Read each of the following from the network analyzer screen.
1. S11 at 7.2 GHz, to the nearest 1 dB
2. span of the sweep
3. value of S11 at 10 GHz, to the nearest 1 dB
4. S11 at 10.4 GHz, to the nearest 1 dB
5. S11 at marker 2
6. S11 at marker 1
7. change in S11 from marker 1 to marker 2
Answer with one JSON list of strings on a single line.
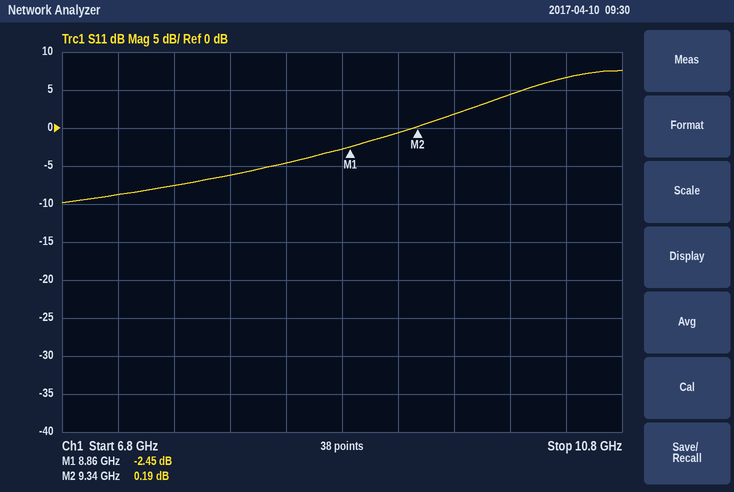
["-9 dB", "4 GHz", "4 dB", "7 dB", "0.19 dB", "-2.45 dB", "2.64 dB"]
